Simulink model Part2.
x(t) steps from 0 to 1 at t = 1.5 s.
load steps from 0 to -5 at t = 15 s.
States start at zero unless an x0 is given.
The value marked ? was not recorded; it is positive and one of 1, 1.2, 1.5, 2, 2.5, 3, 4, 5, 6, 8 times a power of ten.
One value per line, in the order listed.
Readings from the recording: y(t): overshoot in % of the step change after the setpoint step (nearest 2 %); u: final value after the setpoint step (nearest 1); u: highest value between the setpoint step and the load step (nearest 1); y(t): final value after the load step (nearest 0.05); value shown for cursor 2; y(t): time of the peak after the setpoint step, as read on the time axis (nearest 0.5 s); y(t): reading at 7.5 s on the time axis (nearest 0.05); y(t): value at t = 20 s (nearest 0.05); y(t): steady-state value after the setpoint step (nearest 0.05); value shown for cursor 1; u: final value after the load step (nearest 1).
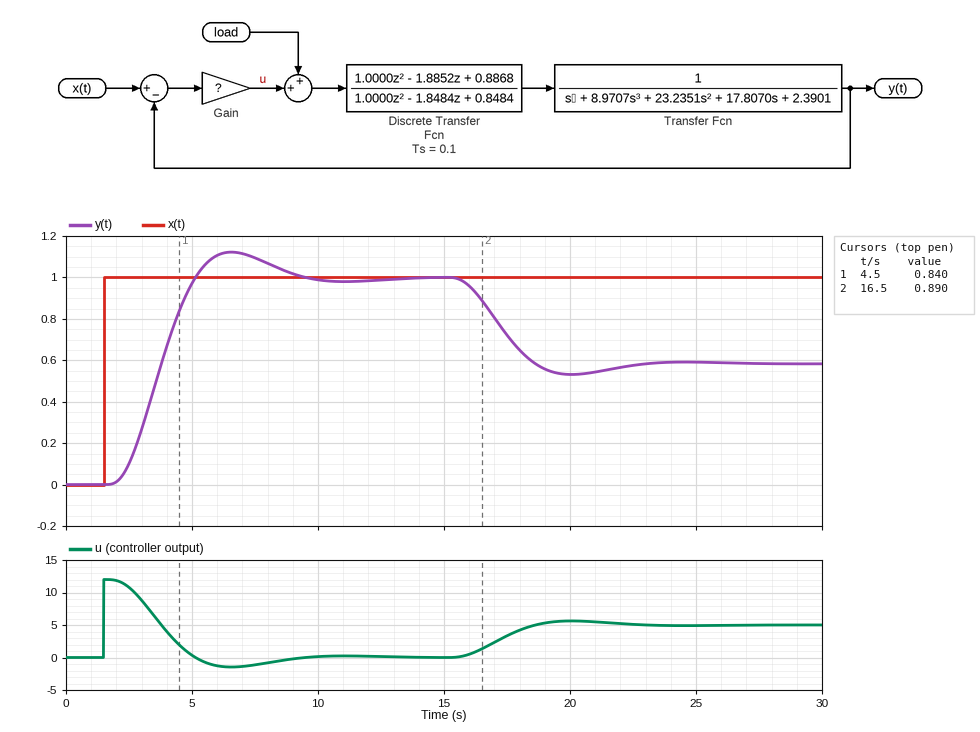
12 %
0
12
0.60
0.890
6.5 s
1.10
0.55
1.00
0.840
5
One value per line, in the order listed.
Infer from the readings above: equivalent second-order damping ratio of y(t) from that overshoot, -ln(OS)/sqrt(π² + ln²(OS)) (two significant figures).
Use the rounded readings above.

0.56
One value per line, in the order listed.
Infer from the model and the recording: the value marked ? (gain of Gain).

12
